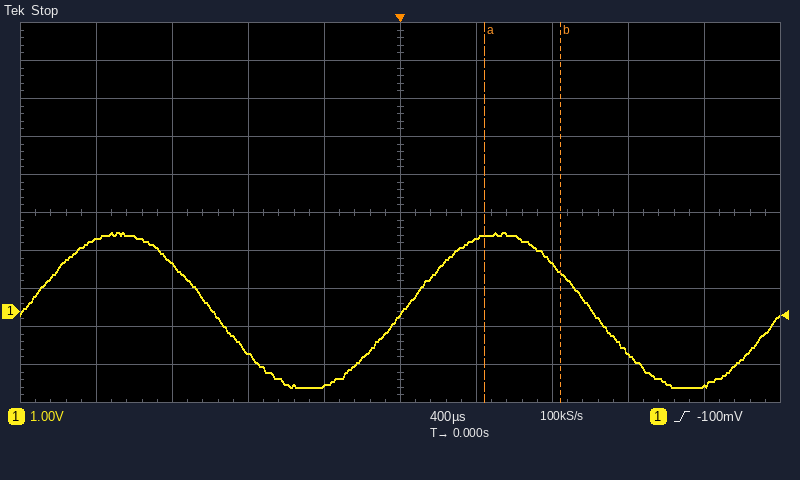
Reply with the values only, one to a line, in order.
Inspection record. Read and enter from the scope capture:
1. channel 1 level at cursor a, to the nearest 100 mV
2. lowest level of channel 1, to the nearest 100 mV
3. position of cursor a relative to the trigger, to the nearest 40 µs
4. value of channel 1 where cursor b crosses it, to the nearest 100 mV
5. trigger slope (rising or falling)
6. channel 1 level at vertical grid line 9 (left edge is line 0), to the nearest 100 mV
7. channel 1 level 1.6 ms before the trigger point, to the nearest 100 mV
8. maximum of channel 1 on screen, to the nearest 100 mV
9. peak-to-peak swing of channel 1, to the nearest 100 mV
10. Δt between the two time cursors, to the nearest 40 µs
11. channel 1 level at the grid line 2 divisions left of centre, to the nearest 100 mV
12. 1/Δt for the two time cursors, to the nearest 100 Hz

2.0 V
-2.0 V
+440 µs
1.0 V
rising
-1.9 V
1.9 V
2.1 V
4.1 V
400 µs
-1.1 V
2.5 kHz
